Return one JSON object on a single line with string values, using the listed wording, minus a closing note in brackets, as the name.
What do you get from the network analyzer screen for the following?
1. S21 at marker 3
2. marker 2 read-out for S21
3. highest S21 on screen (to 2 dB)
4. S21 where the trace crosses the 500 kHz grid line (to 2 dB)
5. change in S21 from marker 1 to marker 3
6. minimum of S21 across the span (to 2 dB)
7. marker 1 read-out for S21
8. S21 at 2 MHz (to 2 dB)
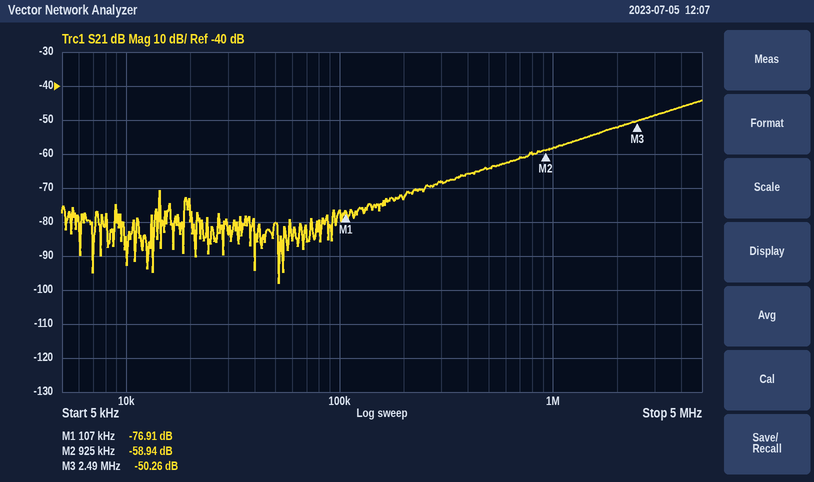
{"S21 at marker 3": "-50.26 dB", "marker 2 read-out for S21": "-58.94 dB", "highest S21 on screen": "-44 dB", "S21 where the trace crosses the 500 kHz grid line": "-64 dB", "change in S21 from marker 1 to marker 3": "26.65 dB", "minimum of S21 across the span": "-98 dB", "marker 1 read-out for S21": "-76.91 dB", "S21 at 2 MHz": "-52 dB"}
